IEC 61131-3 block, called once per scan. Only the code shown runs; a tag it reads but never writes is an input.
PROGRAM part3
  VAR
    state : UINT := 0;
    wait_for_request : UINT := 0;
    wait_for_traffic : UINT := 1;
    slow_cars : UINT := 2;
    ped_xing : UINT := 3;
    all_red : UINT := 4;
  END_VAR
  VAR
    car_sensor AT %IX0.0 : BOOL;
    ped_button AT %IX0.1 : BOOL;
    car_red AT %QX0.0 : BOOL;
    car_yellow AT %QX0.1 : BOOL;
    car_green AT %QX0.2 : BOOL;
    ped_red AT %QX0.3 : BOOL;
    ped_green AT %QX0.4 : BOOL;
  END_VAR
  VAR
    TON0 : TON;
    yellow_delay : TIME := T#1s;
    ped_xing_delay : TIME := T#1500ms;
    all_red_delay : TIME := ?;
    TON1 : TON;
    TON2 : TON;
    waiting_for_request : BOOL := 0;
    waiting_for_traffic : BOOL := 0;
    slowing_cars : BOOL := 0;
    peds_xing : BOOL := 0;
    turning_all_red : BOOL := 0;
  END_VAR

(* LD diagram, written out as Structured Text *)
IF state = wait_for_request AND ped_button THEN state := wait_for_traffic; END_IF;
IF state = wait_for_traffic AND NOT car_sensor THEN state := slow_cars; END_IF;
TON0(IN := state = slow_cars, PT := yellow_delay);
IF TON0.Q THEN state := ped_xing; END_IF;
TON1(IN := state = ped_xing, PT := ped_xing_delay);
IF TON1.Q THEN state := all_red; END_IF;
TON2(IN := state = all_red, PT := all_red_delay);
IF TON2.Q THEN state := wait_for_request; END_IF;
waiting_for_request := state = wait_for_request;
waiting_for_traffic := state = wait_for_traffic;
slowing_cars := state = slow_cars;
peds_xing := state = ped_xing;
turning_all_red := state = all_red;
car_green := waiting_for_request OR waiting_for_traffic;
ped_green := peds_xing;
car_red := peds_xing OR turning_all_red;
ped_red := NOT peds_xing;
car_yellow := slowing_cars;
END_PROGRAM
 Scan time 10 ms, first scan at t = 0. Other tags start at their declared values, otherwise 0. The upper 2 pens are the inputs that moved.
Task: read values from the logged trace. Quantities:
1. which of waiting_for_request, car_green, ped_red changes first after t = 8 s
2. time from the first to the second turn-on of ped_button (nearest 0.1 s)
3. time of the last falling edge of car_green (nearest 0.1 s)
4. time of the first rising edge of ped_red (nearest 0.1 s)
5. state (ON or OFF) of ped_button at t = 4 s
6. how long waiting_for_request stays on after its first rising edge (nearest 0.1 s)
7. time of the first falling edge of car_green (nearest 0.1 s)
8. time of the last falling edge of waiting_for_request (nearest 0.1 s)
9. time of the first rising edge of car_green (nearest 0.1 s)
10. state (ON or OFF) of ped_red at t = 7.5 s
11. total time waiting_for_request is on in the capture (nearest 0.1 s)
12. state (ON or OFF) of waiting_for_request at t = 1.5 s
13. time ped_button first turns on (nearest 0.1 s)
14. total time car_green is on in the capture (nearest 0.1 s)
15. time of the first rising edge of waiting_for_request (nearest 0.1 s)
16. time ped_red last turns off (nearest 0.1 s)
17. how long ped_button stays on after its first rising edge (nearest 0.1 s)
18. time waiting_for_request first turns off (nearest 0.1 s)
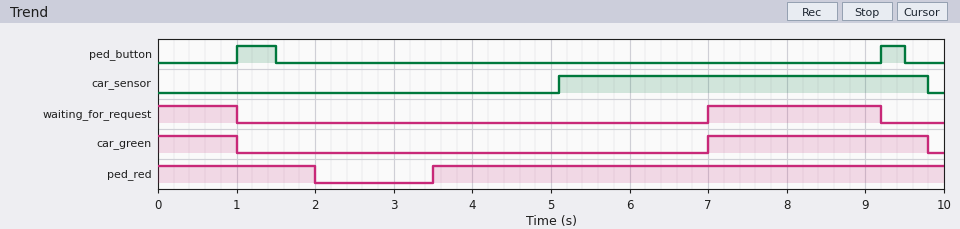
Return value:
waiting_for_request
8.2 s
9.8 s
3.5 s
OFF
2.2 s
1.0 s
9.2 s
7.0 s
ON
3.2 s
OFF
1.0 s
3.8 s
7.0 s
2.0 s
0.5 s
1.0 s
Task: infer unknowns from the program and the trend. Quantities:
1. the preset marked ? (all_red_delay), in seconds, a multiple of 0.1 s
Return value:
3.5 s
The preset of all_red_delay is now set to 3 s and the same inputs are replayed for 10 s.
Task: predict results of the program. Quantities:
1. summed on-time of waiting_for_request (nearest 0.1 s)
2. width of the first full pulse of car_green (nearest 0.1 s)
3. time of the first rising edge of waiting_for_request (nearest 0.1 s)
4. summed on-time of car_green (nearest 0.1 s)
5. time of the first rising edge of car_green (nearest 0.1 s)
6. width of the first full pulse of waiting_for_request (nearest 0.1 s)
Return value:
3.7 s
3.3 s
6.5 s
4.3 s
6.5 s
2.7 s
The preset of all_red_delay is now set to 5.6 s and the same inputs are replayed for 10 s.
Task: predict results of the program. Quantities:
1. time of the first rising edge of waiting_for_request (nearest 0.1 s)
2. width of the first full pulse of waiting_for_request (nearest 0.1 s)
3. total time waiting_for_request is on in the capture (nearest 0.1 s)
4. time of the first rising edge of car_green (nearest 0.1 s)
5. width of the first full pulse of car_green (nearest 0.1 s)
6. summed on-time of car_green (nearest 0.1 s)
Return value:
9.1 s
0.1 s
1.1 s
9.1 s
0.7 s
1.7 s
